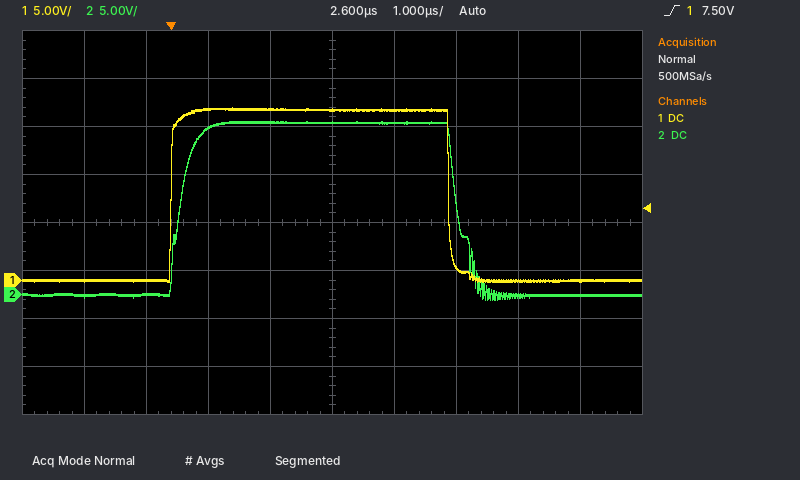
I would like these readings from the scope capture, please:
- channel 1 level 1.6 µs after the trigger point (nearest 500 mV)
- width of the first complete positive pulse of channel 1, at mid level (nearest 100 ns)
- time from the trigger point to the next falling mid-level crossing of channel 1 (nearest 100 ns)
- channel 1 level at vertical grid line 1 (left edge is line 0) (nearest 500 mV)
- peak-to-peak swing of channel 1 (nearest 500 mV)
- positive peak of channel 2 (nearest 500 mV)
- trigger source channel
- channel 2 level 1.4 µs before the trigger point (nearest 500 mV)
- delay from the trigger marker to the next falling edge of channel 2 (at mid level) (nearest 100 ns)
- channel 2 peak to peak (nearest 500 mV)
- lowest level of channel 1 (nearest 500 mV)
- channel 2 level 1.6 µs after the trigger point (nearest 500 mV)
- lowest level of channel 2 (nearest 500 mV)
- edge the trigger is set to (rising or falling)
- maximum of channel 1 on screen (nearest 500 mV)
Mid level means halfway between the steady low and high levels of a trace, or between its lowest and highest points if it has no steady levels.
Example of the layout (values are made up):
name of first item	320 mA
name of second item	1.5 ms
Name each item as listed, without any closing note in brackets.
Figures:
channel 1 level 1.6 µs after the trigger point	18.0 V
width of the first complete positive pulse of channel 1, at mid level	4.5 µs
time from the trigger point to the next falling mid-level crossing of channel 1	4.5 µs
channel 1 level at vertical grid line 1 (left edge is line 0)	0.0 V
peak-to-peak swing of channel 1	18.0 V
positive peak of channel 2	18.0 V
trigger source channel	channel 1
channel 2 level 1.4 µs before the trigger point	0.0 V
delay from the trigger marker to the next falling edge of channel 2 (at mid level)	4.6 µs
channel 2 peak to peak	18.5 V
lowest level of channel 1	0.0 V
channel 2 level 1.6 µs after the trigger point	18.0 V
lowest level of channel 2	-500 mV
edge the trigger is set to	rising
maximum of channel 1 on screen	18.0 V
